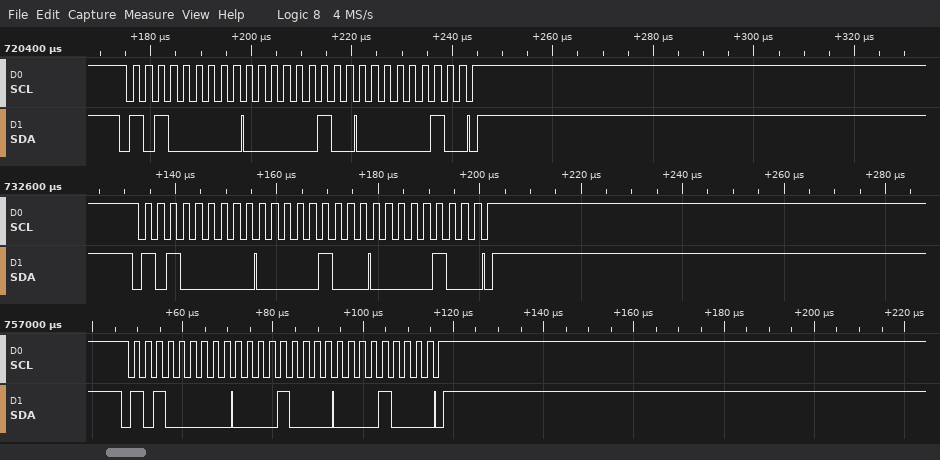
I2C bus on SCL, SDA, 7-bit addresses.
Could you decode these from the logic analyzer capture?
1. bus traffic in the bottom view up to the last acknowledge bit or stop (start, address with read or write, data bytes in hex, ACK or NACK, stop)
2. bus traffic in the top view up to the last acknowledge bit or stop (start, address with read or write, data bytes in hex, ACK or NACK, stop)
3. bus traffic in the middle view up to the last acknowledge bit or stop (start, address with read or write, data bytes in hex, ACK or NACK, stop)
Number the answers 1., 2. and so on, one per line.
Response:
1. start, address 50 write ACK, 08 ACK, 08 ACK, stop
2. start, address 50 write ACK, 02 ACK, 02 ACK, stop
3. start, address 50 write ACK, 04 ACK, 04 ACK, stop
